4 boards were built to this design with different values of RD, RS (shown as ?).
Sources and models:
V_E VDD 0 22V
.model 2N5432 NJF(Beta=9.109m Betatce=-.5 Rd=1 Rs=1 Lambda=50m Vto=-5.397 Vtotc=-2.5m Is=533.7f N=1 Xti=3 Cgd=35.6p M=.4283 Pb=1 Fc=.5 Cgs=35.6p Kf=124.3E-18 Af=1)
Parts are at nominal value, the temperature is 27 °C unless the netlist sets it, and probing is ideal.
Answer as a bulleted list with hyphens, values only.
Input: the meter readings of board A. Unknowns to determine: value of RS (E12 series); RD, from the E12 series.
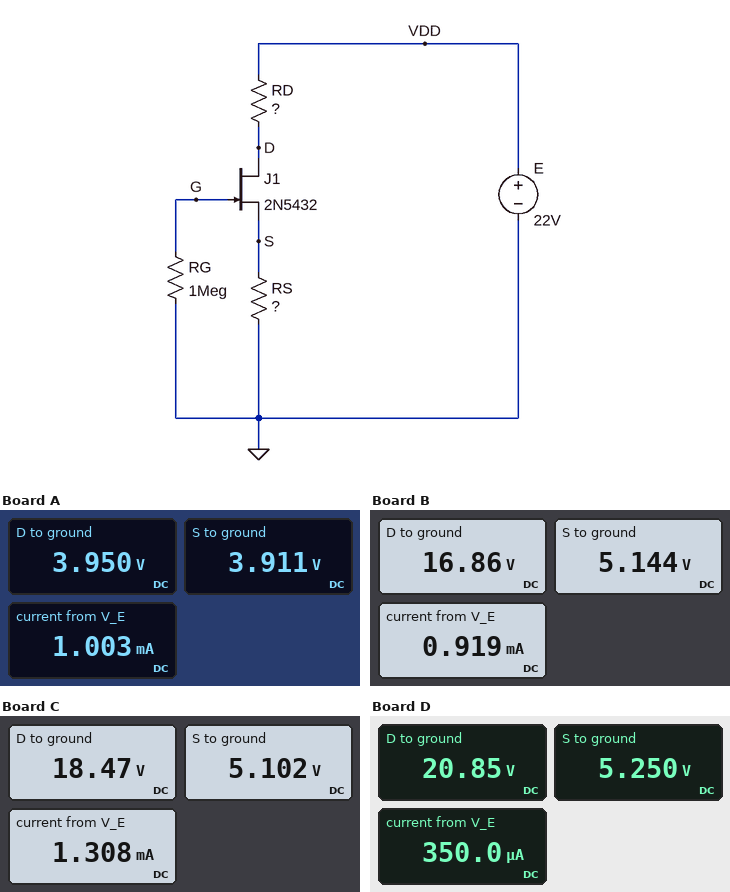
- 3.9 kΩ
- 18 kΩ
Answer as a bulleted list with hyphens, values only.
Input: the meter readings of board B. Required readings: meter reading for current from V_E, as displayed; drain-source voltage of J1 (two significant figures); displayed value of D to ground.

- 0.919 mA
- 12 V
- 16.86 V
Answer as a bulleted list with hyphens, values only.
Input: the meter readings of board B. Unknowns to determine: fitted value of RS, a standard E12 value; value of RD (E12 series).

- 5.6 kΩ
- 5.6 kΩ
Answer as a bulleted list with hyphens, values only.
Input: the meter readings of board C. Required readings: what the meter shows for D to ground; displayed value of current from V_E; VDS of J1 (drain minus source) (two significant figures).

- 18.47 V
- 1.308 mA
- 13 V
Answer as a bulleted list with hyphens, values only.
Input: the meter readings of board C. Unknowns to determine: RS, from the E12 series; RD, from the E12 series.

- 3.9 kΩ
- 2.7 kΩ
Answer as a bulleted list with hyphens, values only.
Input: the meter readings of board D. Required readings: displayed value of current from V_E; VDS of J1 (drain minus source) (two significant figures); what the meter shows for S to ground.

- 350.0 µA
- 16 V
- 5.250 V
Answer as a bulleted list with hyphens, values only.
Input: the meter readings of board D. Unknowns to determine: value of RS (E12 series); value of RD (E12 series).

- 15 kΩ
- 3.3 kΩ
